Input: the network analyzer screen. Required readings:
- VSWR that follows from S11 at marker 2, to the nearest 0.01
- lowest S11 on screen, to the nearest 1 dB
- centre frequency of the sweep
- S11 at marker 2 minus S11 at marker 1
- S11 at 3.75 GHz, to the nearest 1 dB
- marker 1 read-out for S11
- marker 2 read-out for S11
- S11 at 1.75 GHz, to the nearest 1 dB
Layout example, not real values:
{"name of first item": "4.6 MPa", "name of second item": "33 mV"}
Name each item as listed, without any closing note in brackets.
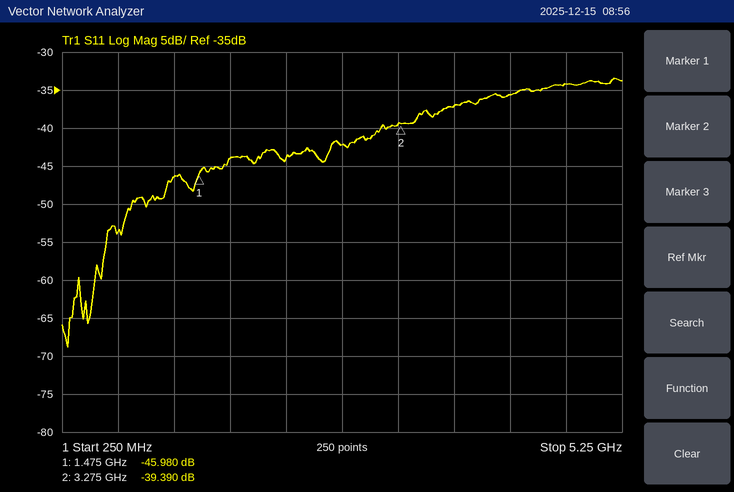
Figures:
{"VSWR that follows from S11 at marker 2, to the nearest 0.01": "1.02", "lowest S11 on screen, to the nearest 1 dB": "-69 dB", "centre frequency of the sweep": "2.75 GHz", "S11 at marker 2 minus S11 at marker 1": "6.590 dB", "S11 at 3.75 GHz, to the nearest 1 dB": "-37 dB", "marker 1 read-out for S11": "-45.980 dB", "marker 2 read-out for S11": "-39.390 dB", "S11 at 1.75 GHz, to the nearest 1 dB": "-44 dB"}
